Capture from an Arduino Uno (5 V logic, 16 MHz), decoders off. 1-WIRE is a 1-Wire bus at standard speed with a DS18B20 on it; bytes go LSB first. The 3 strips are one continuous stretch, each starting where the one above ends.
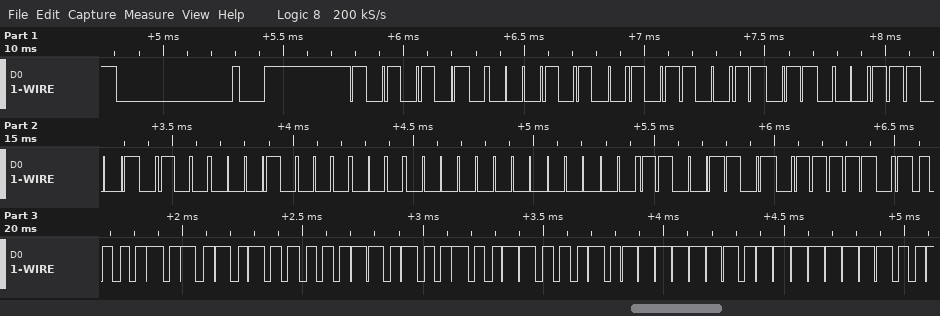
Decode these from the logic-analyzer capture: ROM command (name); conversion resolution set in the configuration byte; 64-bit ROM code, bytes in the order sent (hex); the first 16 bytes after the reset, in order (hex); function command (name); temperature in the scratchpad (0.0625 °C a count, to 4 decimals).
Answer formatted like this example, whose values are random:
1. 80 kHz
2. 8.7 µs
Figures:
1. Match ROM
2. 12 bits
3. 28 CD C6 29 08 00 00 B3
4. 55 28 CD C6 29 08 00 00 B3 BE 50 05 4B 46 7F FF
5. Read Scratchpad
6. 85.0000 °C
